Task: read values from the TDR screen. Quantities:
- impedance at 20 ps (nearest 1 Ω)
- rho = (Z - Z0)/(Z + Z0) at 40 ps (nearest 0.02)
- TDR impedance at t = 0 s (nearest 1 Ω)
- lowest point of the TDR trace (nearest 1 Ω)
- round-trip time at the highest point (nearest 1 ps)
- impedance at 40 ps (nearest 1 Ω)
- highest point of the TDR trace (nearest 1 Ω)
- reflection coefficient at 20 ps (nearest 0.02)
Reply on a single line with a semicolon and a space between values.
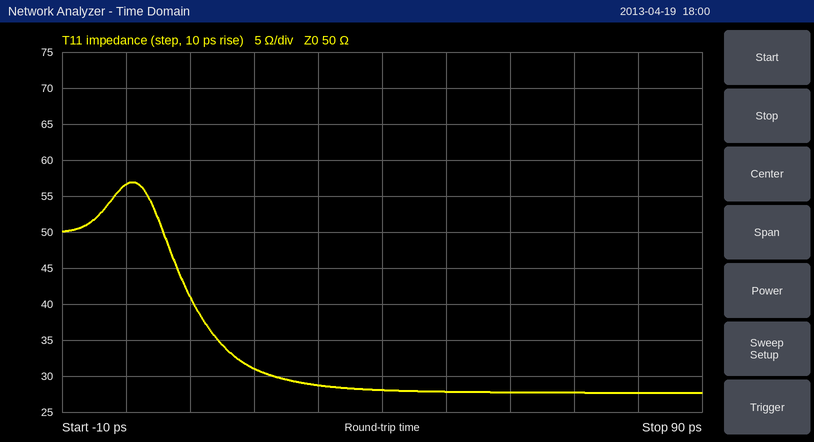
31 Ω; -0.28; 57 Ω; 28 Ω; 1 ps; 28 Ω; 57 Ω; -0.24
